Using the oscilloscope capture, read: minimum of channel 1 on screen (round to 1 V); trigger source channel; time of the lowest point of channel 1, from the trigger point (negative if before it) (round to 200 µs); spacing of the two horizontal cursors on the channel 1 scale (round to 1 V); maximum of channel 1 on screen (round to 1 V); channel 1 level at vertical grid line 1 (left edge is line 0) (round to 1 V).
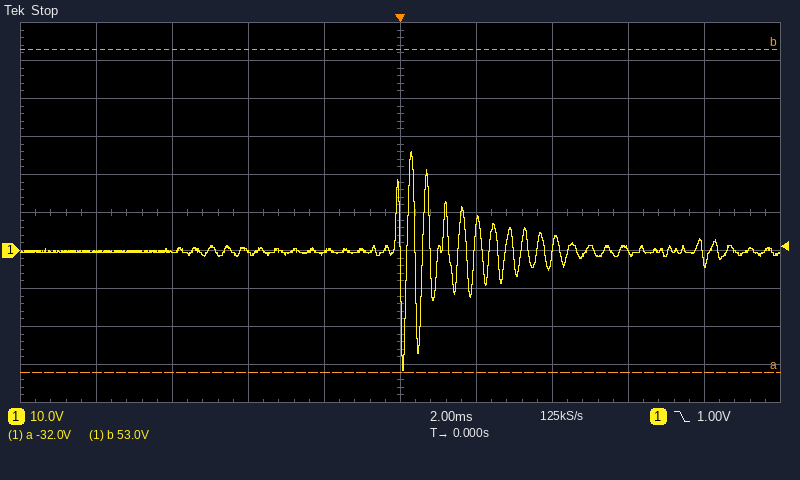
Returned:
-32 V
channel 1
0.0 ms
85 V
26 V
0 V
